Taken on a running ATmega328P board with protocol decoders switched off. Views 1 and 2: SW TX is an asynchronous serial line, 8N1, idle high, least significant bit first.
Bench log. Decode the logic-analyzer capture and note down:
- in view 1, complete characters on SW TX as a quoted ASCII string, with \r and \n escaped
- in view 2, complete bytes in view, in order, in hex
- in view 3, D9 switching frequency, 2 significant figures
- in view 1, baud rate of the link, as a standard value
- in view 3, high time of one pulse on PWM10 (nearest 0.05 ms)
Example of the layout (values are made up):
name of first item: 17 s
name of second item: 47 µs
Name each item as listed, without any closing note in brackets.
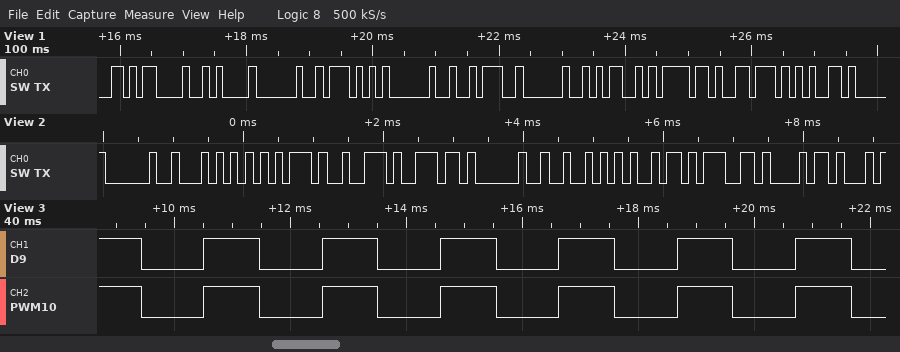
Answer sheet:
in view 1, complete characters on SW TX as a quoted ASCII string, with \r and \n escaped: "\r\n W : Move"
in view 2, complete bytes in view, in order, in hex: 20 54 75 72 6E 20 52 69 67 68
in view 3, D9 switching frequency, 2 significant figures: 490 Hz
in view 1, baud rate of the link, as a standard value: 9600 baud
in view 3, high time of one pulse on PWM10: 0.95 ms
